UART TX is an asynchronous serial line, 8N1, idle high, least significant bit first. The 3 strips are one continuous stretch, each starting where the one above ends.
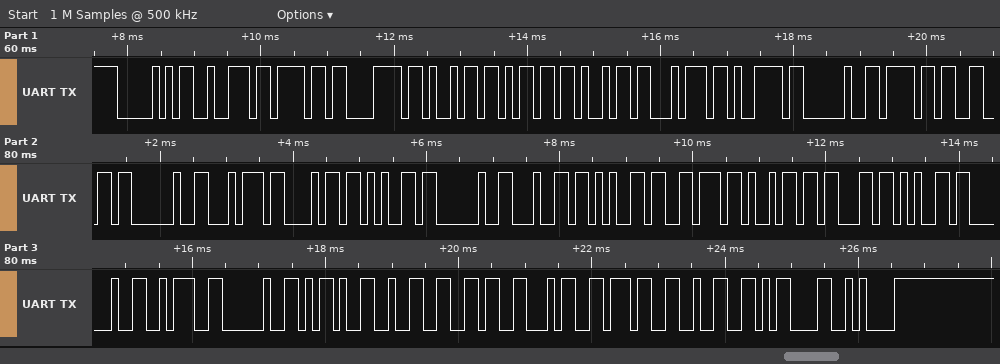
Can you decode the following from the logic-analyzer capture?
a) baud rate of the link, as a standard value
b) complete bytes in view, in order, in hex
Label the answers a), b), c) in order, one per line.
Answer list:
a) 9600 baud
b) 50 72 6F 78 69 6D 69 74 79 20 6F 66 20 74 68 65 20 64 65 76 69 63 65 20 3A 20 2D 32 36 34 37 32 0D 0A
